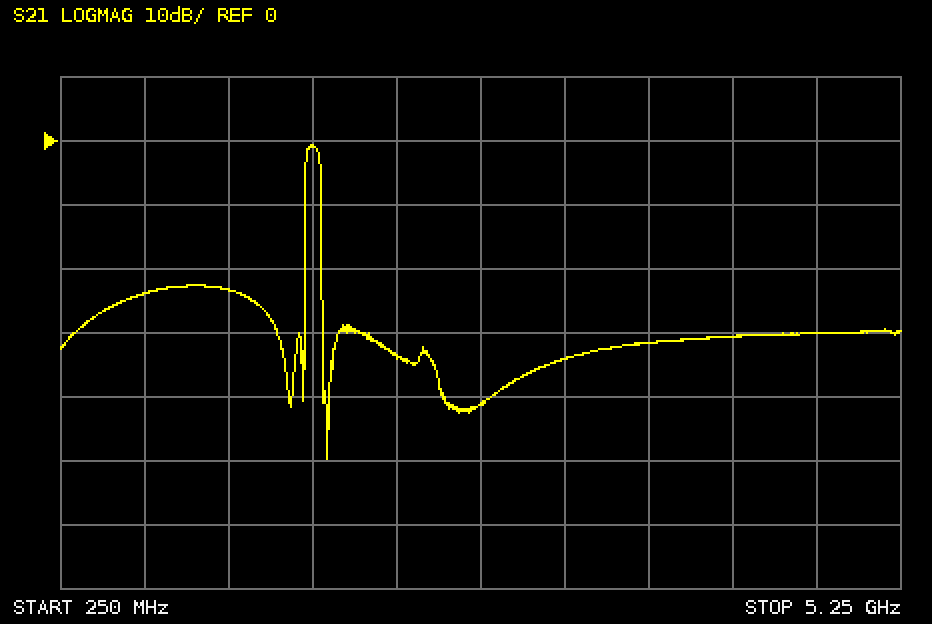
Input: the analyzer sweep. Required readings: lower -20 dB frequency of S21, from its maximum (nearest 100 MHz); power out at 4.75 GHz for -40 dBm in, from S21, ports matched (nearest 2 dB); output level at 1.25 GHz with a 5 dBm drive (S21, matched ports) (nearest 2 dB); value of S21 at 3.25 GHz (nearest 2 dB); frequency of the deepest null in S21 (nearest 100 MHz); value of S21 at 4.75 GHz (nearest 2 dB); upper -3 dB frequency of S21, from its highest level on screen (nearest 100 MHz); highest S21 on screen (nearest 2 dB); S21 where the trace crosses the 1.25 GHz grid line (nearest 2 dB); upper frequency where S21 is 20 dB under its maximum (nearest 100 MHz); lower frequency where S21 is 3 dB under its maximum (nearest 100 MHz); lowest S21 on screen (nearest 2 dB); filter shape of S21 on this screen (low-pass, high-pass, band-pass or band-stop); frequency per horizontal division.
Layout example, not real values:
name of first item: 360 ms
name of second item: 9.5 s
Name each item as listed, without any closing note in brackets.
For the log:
lower -20 dB frequency of S21, from its maximum: 1.7 GHz
power out at 4.75 GHz for -40 dBm in, from S21, ports matched: -70 dBm
output level at 1.25 GHz with a 5 dBm drive (S21, matched ports): -18 dBm
value of S21 at 3.25 GHz: -34 dB
frequency of the deepest null in S21: 1.8 GHz
value of S21 at 4.75 GHz: -30 dB
upper -3 dB frequency of S21, from its highest level on screen: 1.8 GHz
highest S21 on screen: 0 dB
S21 where the trace crosses the 1.25 GHz grid line: -24 dB
upper frequency where S21 is 20 dB under its maximum: 1.8 GHz
lower frequency where S21 is 3 dB under its maximum: 1.7 GHz
lowest S21 on screen: -50 dB
filter shape of S21 on this screen: band-pass
frequency per horizontal division: 500 MHz
